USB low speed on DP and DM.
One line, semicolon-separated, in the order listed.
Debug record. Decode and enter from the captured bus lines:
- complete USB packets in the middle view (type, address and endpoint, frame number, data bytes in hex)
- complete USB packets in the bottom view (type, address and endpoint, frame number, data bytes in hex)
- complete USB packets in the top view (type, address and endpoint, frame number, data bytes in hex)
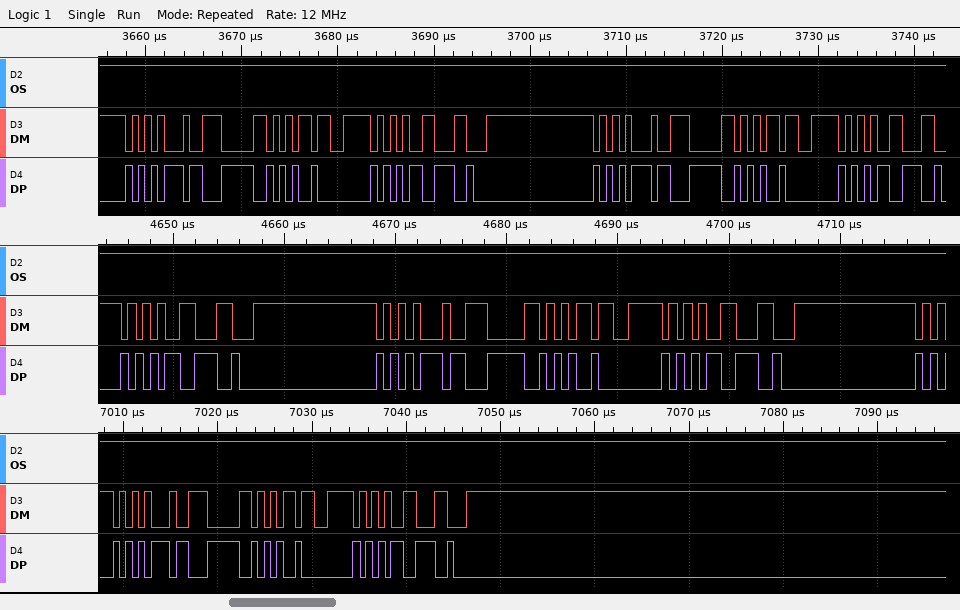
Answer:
NAK, IN ADDR 47 EP 0, NAK; IN ADDR 47 EP 0, NAK; IN ADDR 47 EP 0, NAK, IN ADDR 47 EP 0
